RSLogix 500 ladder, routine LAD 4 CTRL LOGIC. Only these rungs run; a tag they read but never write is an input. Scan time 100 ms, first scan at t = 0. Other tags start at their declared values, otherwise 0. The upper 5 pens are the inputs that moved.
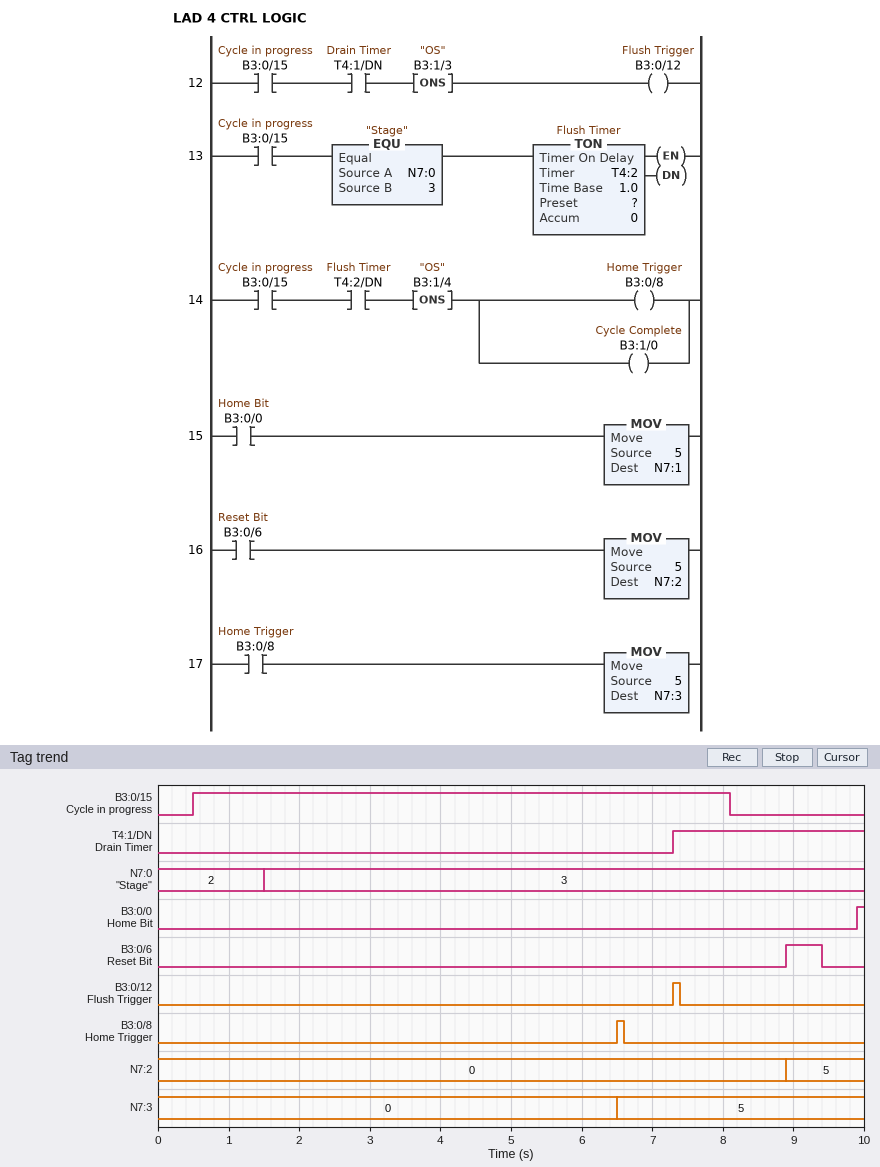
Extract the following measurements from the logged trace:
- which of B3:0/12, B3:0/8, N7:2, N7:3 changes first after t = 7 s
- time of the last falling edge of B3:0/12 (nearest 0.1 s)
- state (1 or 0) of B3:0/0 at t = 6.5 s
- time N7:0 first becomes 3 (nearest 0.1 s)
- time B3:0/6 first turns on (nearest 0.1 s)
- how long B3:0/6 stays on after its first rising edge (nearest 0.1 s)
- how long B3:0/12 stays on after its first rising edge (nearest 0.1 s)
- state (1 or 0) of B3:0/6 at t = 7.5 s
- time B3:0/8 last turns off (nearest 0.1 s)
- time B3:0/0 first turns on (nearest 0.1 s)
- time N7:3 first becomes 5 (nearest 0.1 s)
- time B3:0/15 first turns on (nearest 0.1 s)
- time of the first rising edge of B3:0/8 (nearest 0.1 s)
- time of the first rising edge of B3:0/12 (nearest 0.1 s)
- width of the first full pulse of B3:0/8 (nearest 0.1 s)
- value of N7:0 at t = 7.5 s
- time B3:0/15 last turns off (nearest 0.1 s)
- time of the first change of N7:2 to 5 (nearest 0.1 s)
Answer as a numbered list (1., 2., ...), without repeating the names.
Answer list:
1. B3:0/12
2. 7.4 s
3. 0
4. 1.5 s
5. 8.9 s
6. 0.5 s
7. 0.1 s
8. 0
9. 6.6 s
10. 9.9 s
11. 6.5 s
12. 0.5 s
13. 6.5 s
14. 7.3 s
15. 0.1 s
16. 3
17. 8.1 s
18. 8.9 s
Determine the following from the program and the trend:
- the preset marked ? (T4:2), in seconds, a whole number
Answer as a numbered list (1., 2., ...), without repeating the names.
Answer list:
1. 5 s
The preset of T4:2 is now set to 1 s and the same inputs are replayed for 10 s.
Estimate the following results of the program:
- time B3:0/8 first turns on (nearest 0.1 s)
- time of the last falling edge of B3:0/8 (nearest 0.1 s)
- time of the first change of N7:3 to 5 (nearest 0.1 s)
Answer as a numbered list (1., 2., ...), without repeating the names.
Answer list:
1. 2.5 s
2. 2.6 s
3. 2.5 s
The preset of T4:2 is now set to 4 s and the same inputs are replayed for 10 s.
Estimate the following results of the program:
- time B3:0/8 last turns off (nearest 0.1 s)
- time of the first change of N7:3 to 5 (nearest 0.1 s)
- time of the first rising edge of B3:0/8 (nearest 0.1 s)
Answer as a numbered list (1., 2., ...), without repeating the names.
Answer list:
1. 5.6 s
2. 5.5 s
3. 5.5 s
